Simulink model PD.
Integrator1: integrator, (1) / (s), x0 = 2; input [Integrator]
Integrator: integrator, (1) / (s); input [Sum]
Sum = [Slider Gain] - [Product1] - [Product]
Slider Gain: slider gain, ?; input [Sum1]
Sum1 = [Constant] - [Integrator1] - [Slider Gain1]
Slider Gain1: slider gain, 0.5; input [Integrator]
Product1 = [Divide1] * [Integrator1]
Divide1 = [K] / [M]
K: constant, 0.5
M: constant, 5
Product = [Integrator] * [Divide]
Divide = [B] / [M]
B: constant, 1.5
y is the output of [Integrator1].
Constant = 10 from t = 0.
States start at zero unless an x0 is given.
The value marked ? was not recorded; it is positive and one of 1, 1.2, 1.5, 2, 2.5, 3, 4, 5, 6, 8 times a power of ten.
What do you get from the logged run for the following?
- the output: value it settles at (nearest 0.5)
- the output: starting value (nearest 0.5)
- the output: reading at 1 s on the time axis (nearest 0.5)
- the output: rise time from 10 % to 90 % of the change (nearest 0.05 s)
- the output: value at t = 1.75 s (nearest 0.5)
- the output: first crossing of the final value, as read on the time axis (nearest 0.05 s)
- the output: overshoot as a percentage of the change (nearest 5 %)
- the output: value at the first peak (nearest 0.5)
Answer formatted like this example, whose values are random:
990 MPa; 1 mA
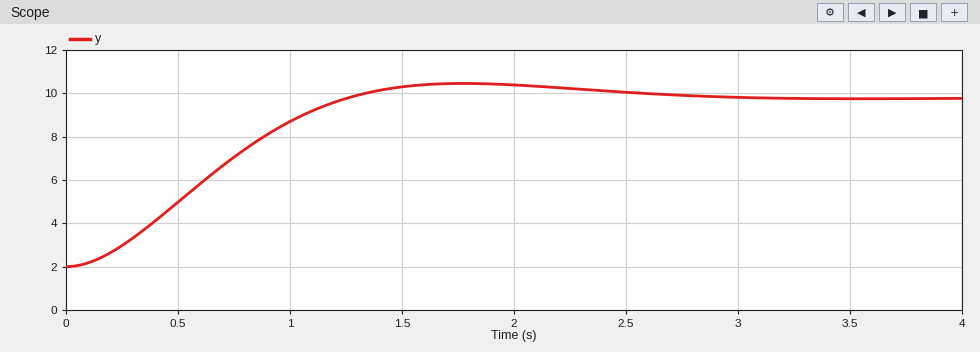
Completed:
10.0; 2.0; 8.5; 0.85 s; 10.5; 1.25 s; 10 %; 10.5
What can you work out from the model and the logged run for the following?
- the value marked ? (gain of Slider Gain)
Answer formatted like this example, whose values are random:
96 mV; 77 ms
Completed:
5
